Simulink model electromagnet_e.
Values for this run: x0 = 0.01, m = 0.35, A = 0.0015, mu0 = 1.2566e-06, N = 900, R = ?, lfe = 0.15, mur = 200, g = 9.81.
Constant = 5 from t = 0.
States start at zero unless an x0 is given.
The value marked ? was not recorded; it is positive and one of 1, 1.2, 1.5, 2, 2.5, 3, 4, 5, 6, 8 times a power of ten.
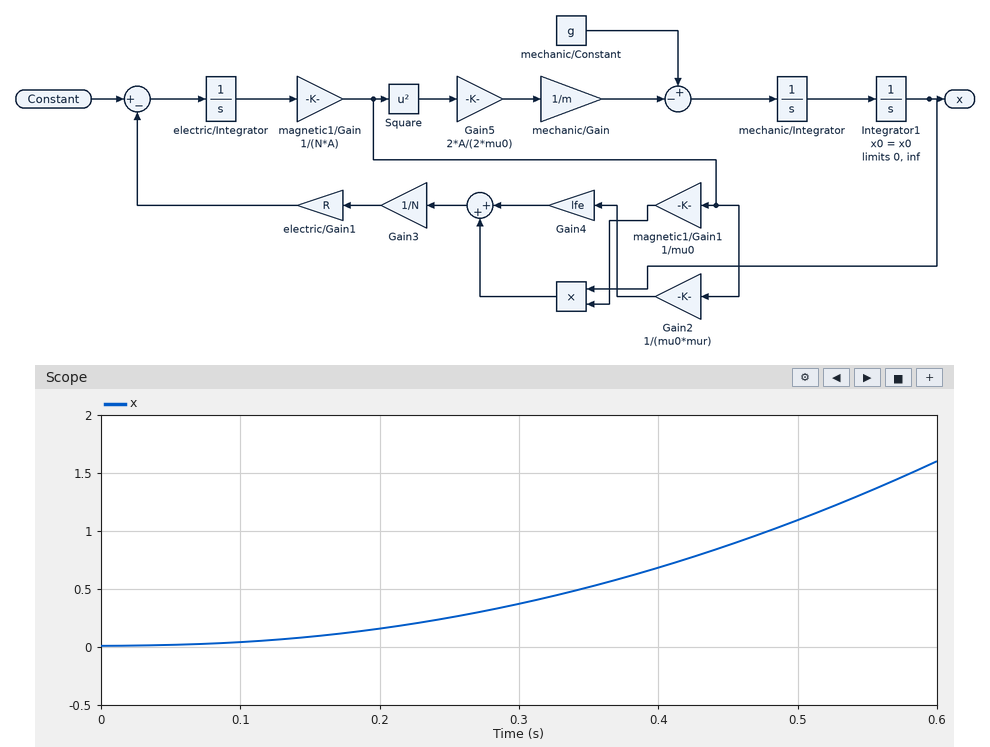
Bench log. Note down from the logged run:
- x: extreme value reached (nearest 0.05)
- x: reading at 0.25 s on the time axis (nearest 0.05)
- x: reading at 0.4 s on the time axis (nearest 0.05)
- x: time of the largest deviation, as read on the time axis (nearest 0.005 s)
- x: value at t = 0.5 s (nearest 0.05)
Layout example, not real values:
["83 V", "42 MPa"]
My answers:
["1.60", "0.25", "0.70", "0.600 s", "1.10"]
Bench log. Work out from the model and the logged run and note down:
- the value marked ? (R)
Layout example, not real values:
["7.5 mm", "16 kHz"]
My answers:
["10"]
